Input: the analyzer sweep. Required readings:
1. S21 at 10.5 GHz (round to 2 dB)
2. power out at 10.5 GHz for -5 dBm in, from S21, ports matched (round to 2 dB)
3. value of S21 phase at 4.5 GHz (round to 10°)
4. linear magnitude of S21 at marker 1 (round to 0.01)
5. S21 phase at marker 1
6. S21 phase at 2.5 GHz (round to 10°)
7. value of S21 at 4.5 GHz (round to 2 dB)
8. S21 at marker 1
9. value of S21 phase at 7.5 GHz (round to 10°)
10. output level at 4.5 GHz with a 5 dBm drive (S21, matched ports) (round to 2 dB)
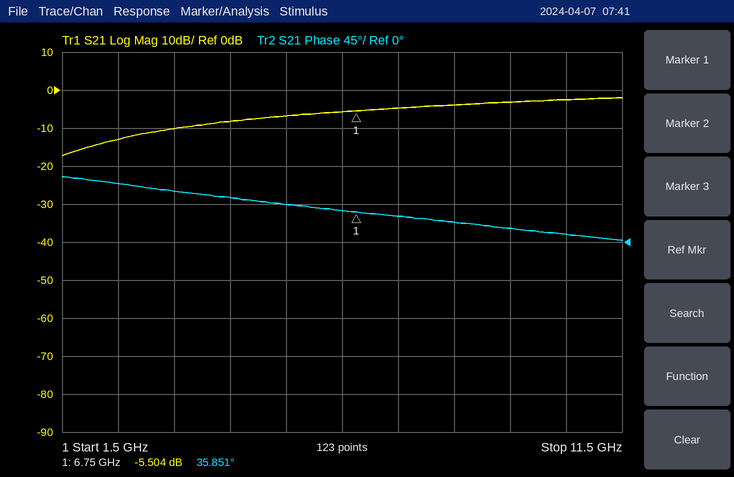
-2 dB
-8 dBm
50°
0.53
35.851°
70°
-8 dB
-5.504 dB
30°
-4 dBm
